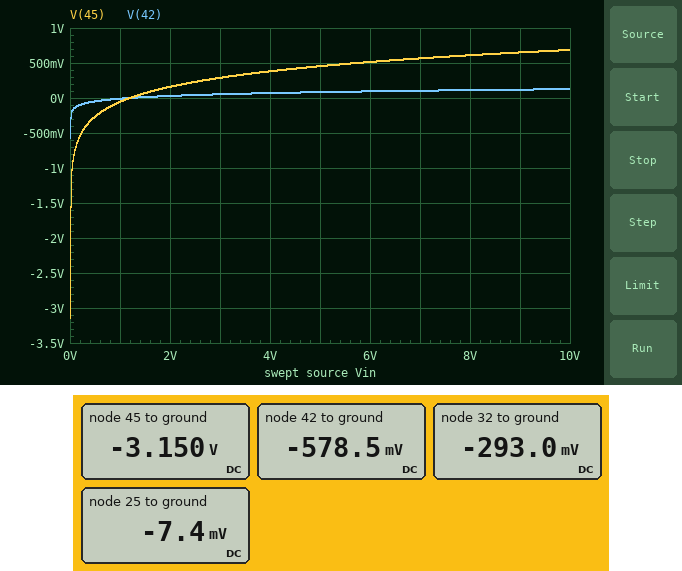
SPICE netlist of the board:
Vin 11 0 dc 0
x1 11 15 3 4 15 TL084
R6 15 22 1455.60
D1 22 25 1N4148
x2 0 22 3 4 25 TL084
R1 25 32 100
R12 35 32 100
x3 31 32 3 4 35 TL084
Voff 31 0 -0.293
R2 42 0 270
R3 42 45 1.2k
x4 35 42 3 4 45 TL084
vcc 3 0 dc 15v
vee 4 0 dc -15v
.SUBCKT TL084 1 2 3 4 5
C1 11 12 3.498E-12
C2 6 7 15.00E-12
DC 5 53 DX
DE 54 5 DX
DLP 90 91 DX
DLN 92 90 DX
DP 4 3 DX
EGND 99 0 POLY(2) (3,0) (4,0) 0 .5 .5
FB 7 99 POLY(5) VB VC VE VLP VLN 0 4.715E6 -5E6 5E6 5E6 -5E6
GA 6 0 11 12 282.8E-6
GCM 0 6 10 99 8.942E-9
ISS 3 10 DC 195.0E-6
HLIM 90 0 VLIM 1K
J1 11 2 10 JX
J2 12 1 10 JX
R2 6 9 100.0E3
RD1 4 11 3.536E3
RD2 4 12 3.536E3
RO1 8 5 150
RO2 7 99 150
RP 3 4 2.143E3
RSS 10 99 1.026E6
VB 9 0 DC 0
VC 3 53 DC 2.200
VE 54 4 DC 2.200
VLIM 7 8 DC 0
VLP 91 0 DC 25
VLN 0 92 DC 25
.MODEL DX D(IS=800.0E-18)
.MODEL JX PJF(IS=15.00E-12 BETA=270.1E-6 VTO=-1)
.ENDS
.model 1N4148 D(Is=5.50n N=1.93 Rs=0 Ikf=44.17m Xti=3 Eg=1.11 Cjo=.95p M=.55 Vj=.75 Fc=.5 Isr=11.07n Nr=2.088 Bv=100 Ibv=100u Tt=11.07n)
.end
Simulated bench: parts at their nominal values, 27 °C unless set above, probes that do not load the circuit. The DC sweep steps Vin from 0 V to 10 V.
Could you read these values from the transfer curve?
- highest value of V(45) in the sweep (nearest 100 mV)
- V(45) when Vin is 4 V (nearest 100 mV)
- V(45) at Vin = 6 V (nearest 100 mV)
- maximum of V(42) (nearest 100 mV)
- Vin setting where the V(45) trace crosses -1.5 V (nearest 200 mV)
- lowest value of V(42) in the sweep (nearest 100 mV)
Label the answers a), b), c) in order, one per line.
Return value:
a) 700 mV
b) 400 mV
c) 500 mV
d) 100 mV
e) 0 V
f) -600 mV
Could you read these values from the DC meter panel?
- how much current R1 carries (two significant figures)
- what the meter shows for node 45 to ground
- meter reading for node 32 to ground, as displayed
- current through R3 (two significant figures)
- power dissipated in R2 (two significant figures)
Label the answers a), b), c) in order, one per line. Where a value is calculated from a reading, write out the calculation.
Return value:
a) (-7.4 mV - (-293 mV)) / 100 Ω = 2.9 mA
b) -3.150 V
c) -293.0 mV
d) (-578.5 mV - (-3.15 V)) / 1.2 kΩ = 2.1 mA
e) (0 V - (-578.5 mV))^2 / 270 Ω = 1.2 mW
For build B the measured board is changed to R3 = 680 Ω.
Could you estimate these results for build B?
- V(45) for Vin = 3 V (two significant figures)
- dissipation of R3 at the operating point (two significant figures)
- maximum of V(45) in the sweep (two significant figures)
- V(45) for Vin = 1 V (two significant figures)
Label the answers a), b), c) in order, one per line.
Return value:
a) 190 mV
b) 3.1 mW
c) 440 mV
d) -36 mV
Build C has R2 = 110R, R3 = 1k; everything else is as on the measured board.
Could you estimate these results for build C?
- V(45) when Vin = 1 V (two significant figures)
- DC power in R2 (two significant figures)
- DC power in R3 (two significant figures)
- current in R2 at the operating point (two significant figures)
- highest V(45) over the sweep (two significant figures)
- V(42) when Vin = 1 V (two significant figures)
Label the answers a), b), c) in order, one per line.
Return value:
a) -100 mV
b) 3.0 mW
c) 28 mW
d) 5.3 mA
e) 1.3 V
f) -10 mV
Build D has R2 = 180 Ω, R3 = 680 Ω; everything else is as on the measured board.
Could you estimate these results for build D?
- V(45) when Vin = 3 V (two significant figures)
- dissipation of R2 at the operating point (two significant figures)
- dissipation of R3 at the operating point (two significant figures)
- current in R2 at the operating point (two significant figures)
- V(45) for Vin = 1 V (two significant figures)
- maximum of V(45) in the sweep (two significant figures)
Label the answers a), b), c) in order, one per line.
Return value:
a) 250 mV
b) 1.9 mW
c) 7.0 mW
d) 3.2 mA
e) -49 mV
f) 600 mV
